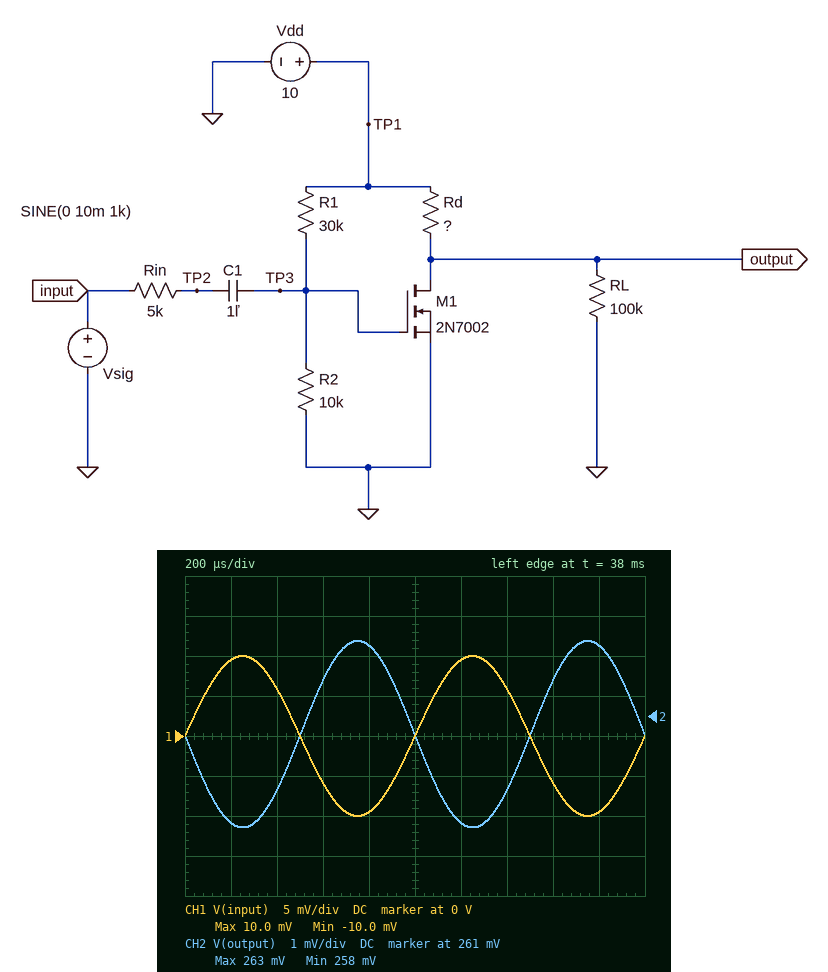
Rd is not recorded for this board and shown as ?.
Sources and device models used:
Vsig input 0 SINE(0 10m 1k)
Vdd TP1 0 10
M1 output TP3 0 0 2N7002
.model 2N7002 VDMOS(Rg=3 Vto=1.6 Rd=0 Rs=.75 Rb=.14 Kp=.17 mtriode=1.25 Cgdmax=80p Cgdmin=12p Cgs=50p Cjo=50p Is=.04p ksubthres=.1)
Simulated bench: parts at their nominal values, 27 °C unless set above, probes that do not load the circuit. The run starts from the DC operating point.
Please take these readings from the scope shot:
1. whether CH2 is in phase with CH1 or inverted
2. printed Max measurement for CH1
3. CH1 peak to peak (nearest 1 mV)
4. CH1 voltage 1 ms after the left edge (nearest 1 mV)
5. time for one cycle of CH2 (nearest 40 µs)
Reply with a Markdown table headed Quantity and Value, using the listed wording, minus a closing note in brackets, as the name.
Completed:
| Quantity | Value |
|---|---|
| whether CH2 is in phase with CH1 or inverted | inverted |
| printed Max measurement for CH1 | 10.0 mV |
| CH1 peak to peak | 20 mV |
| CH1 voltage 1 ms after the left edge | 0 V |
| time for one cycle of CH2 | 1.00 ms |
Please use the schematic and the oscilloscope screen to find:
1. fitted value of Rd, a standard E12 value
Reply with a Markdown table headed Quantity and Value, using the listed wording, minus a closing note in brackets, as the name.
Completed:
| Quantity | Value |
|---|---|
| fitted value of Rd, a standard E12 value | 270 Ω |
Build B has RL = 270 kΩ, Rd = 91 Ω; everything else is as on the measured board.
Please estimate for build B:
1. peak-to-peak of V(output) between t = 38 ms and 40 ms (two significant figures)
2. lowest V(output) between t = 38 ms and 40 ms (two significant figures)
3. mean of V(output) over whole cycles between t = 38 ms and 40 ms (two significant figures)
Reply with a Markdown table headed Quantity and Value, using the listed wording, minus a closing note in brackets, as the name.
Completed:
| Quantity | Value |
|---|---|
| peak-to-peak of V(output) between t = 38 ms and 40 ms | 140 mV |
| lowest V(output) between t = 38 ms and 40 ms | 4.3 V |
| mean of V(output) over whole cycles between t = 38 ms and 40 ms | 4.4 V |
